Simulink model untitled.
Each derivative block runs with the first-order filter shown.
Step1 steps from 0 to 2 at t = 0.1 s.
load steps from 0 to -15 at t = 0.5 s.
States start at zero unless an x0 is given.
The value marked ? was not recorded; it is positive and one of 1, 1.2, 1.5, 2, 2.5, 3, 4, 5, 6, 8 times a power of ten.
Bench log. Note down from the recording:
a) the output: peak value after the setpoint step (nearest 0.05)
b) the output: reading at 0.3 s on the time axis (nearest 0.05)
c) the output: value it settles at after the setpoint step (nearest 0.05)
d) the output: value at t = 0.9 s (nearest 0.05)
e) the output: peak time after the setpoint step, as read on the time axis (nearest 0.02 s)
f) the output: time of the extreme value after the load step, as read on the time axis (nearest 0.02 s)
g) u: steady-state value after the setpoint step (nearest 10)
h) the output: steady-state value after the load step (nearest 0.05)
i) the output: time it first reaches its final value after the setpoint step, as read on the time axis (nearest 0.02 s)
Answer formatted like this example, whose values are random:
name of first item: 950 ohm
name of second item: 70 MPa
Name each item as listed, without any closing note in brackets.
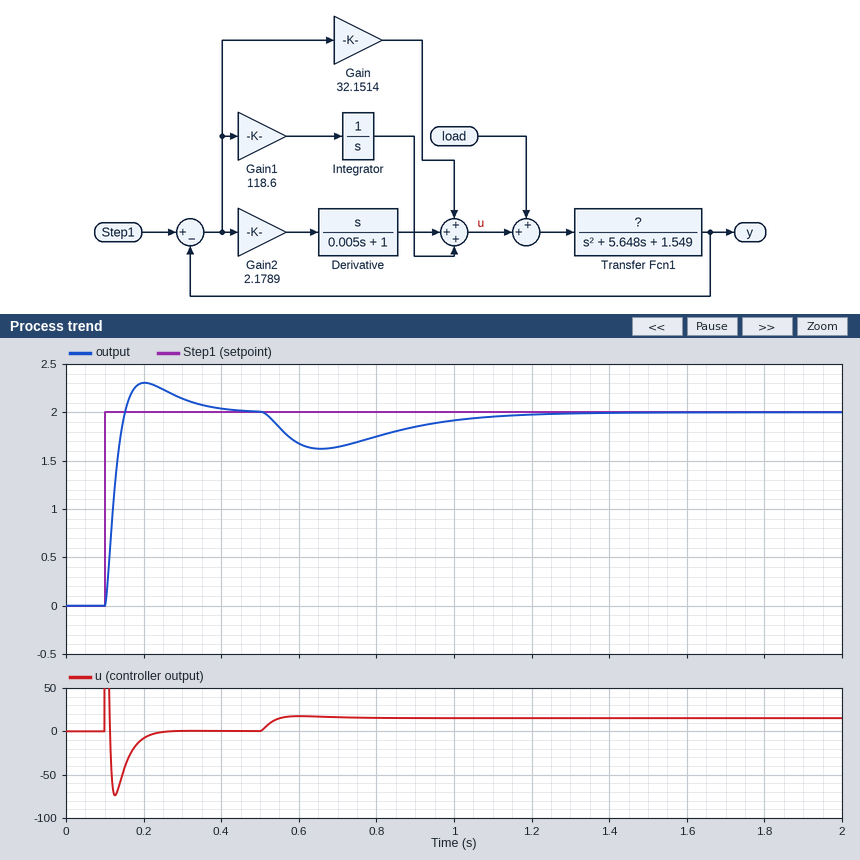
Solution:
the output: peak value after the setpoint step: 2.30
the output: reading at 0.3 s on the time axis: 2.15
the output: value it settles at after the setpoint step: 2.00
the output: value at t = 0.9 s: 1.85
the output: peak time after the setpoint step, as read on the time axis: 0.20 s
the output: time of the extreme value after the load step, as read on the time axis: 0.66 s
u: steady-state value after the setpoint step: 0
the output: steady-state value after the load step: 2.00
the output: time it first reaches its final value after the setpoint step, as read on the time axis: 0.16 s
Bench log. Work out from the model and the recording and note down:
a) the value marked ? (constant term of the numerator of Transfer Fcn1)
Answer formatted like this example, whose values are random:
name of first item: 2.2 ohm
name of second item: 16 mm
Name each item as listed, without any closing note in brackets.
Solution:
the value marked ?: 15
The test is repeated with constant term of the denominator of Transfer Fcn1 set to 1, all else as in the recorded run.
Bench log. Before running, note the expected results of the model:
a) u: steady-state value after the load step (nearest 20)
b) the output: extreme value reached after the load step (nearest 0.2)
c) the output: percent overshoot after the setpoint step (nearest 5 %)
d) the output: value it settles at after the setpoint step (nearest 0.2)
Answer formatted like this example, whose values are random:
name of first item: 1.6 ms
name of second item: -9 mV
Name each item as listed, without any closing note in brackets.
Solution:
u: steady-state value after the load step: 20
the output: extreme value reached after the load step: 1.6
the output: percent overshoot after the setpoint step: 15 %
the output: value it settles at after the setpoint step: 2.0
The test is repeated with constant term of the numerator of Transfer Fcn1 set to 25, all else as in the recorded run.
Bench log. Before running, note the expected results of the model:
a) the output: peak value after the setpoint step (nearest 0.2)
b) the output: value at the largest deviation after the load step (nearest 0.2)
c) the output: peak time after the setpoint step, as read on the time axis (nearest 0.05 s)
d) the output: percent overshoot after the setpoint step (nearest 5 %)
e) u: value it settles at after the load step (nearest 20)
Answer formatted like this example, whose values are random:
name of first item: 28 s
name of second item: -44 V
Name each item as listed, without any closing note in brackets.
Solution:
the output: peak value after the setpoint step: 2.2
the output: value at the largest deviation after the load step: 1.6
the output: peak time after the setpoint step, as read on the time axis: 0.15 s
the output: percent overshoot after the setpoint step: 10 %
u: value it settles at after the load step: 20
